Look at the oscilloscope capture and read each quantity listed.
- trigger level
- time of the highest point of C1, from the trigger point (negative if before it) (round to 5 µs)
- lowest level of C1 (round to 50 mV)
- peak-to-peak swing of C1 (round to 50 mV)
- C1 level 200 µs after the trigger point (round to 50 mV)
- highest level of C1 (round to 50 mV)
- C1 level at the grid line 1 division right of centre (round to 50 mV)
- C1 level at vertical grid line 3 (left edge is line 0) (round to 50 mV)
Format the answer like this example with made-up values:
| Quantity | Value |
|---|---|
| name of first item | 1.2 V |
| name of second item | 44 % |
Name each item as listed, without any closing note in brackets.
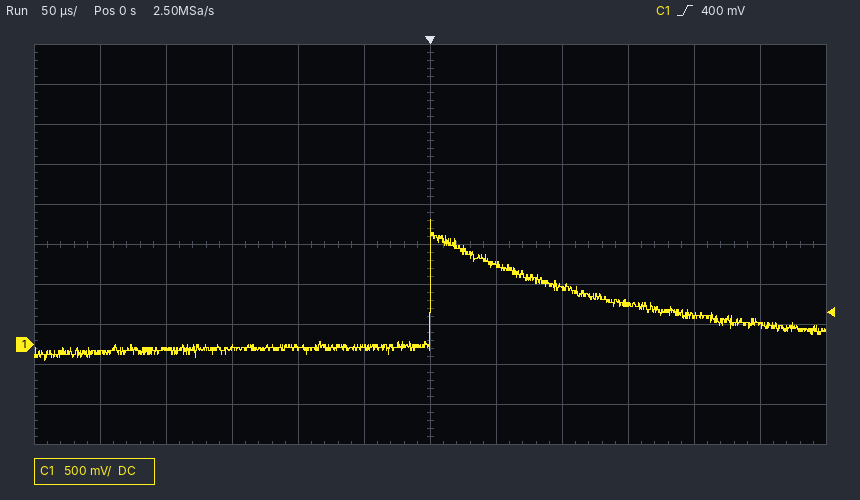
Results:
| Quantity | Value |
|---|---|
| trigger level | 400 mV |
| time of the highest point of C1, from the trigger point (negative if before it) | 0 µs |
| lowest level of C1 | -200 mV |
| peak-to-peak swing of C1 | 1.75 V |
| C1 level 200 µs after the trigger point | 350 mV |
| highest level of C1 | 1.55 V |
| C1 level at the grid line 1 division right of centre | 1.00 V |
| C1 level at vertical grid line 3 (left edge is line 0) | -50 mV |
